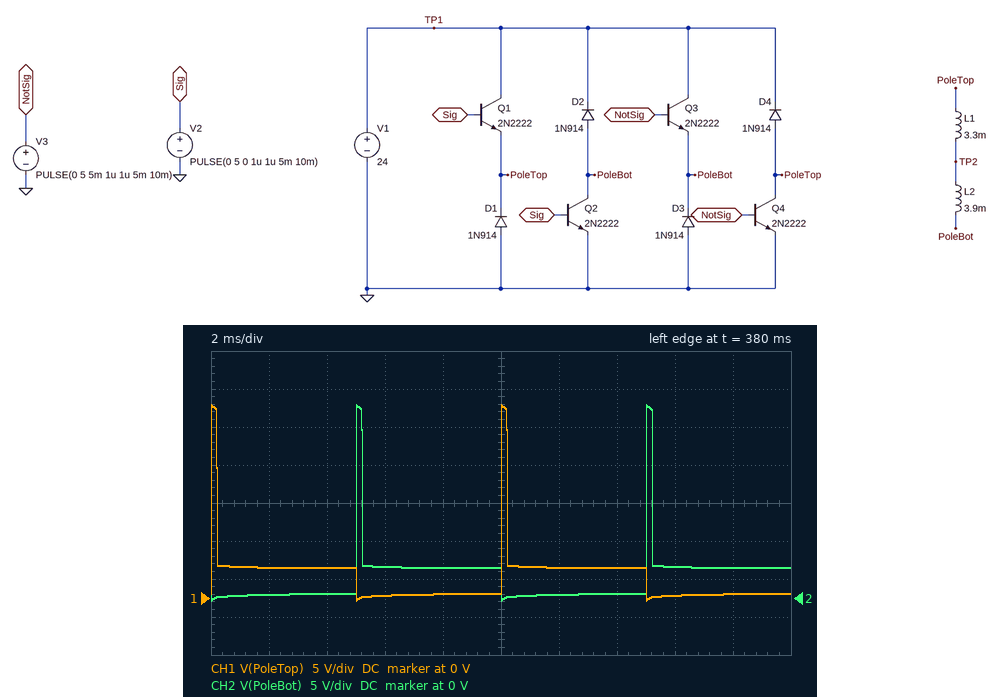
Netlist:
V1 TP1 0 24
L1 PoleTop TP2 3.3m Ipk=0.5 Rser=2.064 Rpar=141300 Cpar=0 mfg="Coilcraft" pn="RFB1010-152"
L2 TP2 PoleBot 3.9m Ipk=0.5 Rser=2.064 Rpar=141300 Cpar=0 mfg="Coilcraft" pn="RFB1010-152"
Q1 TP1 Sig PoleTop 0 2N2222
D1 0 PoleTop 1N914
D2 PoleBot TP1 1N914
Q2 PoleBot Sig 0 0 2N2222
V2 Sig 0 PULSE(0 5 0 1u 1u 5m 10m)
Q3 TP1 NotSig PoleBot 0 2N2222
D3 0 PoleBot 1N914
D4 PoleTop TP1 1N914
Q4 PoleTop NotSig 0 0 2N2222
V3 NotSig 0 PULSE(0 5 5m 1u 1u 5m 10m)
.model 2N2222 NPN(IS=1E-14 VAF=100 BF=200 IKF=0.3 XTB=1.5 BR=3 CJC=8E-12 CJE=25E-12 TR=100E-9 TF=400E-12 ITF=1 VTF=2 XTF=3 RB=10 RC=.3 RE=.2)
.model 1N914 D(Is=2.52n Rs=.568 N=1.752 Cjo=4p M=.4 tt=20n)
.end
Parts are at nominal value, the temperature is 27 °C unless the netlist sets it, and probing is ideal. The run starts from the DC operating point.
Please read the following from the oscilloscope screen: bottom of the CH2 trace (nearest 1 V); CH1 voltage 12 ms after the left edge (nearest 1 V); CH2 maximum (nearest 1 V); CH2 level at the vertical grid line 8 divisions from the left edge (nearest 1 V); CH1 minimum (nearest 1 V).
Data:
0 V
4 V
25 V
4 V
0 V
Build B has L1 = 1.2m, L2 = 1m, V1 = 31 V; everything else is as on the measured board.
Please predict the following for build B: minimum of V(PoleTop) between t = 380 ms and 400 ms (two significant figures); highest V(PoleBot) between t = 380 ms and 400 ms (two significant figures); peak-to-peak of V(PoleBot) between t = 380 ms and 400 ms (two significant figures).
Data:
-340 mV
32 V
33 V
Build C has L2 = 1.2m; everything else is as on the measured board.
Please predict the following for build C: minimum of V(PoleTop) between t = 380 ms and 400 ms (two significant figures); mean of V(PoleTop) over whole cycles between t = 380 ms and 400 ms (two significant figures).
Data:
-340 mV
2.5 V
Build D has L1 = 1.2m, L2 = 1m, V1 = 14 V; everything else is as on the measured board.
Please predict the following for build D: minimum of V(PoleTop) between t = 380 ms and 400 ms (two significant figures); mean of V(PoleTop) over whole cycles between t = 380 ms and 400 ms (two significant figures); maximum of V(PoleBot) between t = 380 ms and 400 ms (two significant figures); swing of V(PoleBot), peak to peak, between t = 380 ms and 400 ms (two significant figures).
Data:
-340 mV
2.3 V
15 V
16 V
